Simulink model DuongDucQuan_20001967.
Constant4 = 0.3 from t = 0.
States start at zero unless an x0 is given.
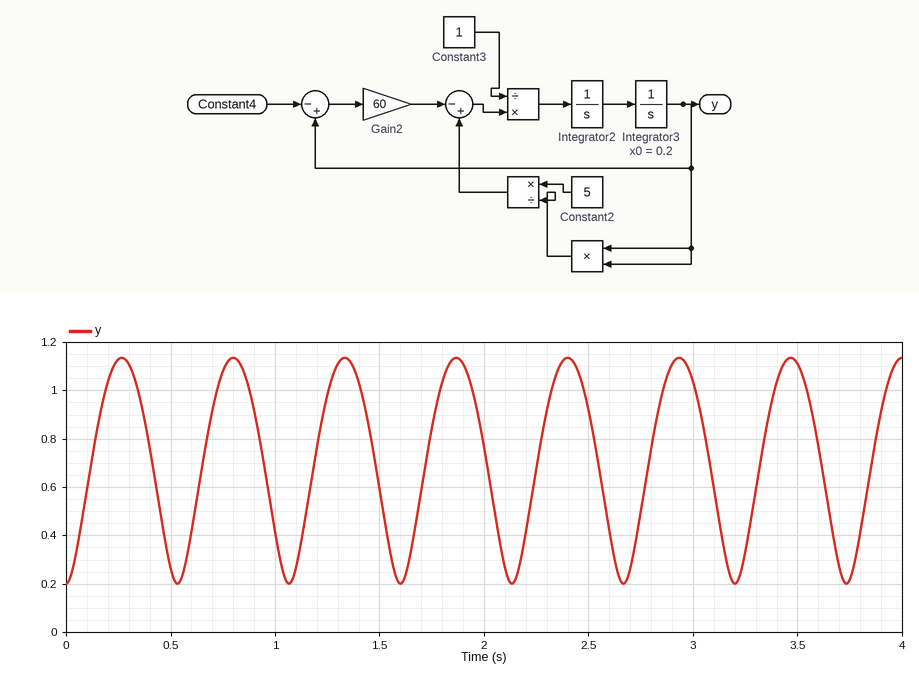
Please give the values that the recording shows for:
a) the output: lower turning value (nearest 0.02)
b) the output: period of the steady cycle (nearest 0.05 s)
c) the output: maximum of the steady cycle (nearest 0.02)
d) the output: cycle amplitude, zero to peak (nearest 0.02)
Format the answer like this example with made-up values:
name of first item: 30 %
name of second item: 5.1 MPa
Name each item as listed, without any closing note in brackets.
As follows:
the output: lower turning value: 0.20
the output: period of the steady cycle: 0.55 s
the output: maximum of the steady cycle: 1.14
the output: cycle amplitude, zero to peak: 0.46
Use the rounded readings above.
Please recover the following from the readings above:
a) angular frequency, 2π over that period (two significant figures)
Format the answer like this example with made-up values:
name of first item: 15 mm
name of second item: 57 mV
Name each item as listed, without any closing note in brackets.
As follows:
angular frequency, 2π over that period: 11 rad/s
